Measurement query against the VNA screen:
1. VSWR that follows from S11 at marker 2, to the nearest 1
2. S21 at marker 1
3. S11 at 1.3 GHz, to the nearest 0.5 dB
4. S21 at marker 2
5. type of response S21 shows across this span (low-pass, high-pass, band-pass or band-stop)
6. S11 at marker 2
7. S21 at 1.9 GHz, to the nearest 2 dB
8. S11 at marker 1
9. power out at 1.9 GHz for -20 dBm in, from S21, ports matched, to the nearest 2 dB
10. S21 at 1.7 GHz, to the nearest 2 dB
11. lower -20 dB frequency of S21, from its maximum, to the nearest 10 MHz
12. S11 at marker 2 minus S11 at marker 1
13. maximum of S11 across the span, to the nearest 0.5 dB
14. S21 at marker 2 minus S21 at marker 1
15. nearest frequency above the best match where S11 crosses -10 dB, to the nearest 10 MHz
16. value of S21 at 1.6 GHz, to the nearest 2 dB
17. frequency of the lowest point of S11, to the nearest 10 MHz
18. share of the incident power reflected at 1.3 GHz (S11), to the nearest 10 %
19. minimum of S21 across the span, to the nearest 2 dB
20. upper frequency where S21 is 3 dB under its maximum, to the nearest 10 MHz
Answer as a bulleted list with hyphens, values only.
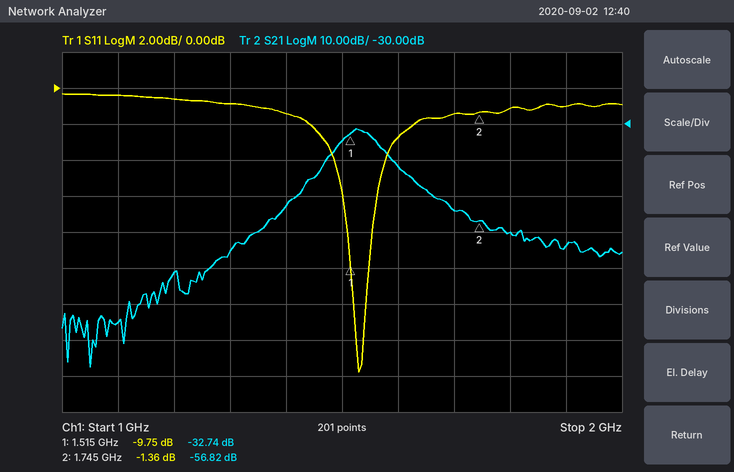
- 13
- -32.74 dB
- -1.0 dB
- -56.82 dB
- band-pass
- -1.36 dB
- -64 dB
- -9.75 dB
- -84 dBm
- -54 dB
- 1.41 GHz
- 8.39 dB
- -0.5 dB
- -24.08 dB
- 1.55 GHz
- -42 dB
- 1.53 GHz
- 80 %
- -98 dB
- 1.56 GHz
